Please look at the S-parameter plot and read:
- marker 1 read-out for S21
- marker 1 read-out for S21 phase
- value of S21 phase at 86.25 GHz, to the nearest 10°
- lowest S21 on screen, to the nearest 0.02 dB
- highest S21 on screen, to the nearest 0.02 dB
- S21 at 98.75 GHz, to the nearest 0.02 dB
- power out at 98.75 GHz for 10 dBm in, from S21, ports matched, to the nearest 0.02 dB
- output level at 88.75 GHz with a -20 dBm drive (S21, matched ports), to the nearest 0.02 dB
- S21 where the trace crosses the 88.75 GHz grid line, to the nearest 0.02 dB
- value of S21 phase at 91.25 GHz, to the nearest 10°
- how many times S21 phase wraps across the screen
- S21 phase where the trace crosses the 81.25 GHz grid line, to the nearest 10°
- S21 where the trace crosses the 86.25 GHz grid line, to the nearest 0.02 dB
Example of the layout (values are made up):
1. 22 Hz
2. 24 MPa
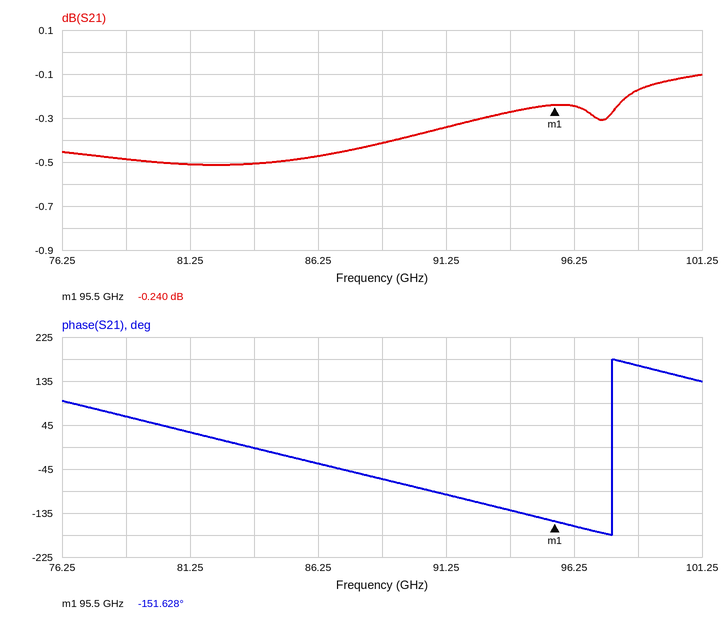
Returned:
1. -0.240 dB
2. -151.628°
3. -30°
4. -0.52 dB
5. -0.10 dB
6. -0.18 dB
7. 9.82 dBm
8. -20.42 dBm
9. -0.42 dB
10. -100°
11. 1
12. 30°
13. -0.48 dB
